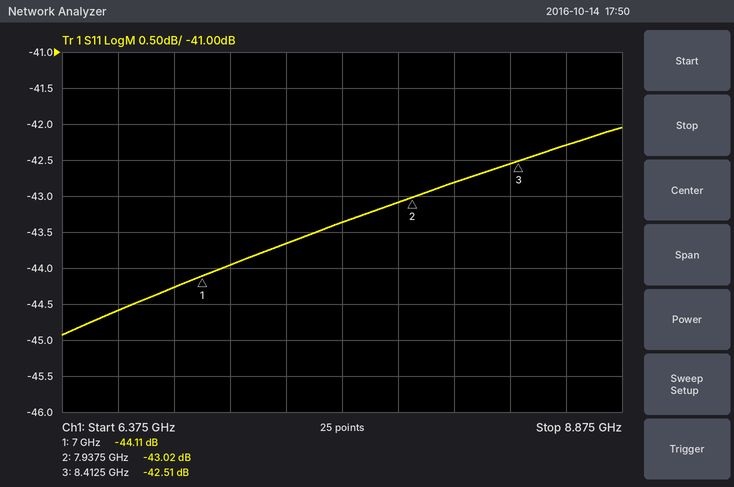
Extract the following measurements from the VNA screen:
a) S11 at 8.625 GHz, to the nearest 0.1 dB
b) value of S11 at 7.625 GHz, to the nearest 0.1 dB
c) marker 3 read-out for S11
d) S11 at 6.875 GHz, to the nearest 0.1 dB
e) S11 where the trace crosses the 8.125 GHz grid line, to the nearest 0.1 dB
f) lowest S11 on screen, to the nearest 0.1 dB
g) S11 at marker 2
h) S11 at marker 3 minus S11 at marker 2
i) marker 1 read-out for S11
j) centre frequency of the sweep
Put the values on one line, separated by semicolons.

-42.3 dB; -43.4 dB; -42.51 dB; -44.3 dB; -42.8 dB; -44.9 dB; -43.02 dB; 0.51 dB; -44.11 dB; 7.625 GHz
